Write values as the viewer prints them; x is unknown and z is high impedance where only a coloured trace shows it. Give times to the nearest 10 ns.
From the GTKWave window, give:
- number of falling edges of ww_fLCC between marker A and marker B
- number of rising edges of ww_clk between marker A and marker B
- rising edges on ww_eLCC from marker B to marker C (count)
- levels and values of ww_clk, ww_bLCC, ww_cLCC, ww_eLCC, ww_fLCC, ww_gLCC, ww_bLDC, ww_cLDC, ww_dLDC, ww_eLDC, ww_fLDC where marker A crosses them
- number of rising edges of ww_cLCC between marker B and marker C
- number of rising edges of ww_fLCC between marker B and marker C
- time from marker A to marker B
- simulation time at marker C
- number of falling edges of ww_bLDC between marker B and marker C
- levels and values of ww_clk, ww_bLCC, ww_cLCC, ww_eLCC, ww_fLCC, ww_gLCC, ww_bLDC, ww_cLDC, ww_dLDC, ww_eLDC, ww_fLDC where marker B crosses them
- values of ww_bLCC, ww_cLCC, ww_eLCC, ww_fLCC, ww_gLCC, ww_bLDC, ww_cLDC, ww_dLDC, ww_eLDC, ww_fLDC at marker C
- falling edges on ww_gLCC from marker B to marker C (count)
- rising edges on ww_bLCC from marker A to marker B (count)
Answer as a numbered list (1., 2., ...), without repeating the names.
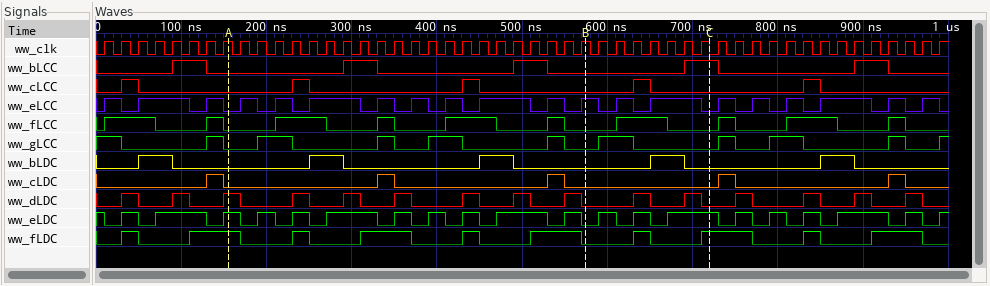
1. 4
2. 21
3. 2
4. ww_clk=1, ww_bLCC=0, ww_cLCC=0, ww_eLCC=0, ww_fLCC=0, ww_gLCC=0, ww_bLDC=0, ww_cLDC=0, ww_dLDC=1, ww_eLDC=1, ww_fLDC=1
5. 1
6. 1
7. 420 ns
8. 720 ns
9. 1
10. ww_clk=1, ww_bLCC=0, ww_cLCC=0, ww_eLCC=1, ww_fLCC=0, ww_gLCC=0, ww_bLDC=0, ww_cLDC=0, ww_dLDC=0, ww_eLDC=0, ww_fLDC=0
11. ww_bLCC=1, ww_cLCC=0, ww_eLCC=0, ww_fLCC=0, ww_gLCC=0, ww_bLDC=0, ww_cLDC=0, ww_dLDC=0, ww_eLDC=1, ww_fLDC=1
12. 1
13. 2
